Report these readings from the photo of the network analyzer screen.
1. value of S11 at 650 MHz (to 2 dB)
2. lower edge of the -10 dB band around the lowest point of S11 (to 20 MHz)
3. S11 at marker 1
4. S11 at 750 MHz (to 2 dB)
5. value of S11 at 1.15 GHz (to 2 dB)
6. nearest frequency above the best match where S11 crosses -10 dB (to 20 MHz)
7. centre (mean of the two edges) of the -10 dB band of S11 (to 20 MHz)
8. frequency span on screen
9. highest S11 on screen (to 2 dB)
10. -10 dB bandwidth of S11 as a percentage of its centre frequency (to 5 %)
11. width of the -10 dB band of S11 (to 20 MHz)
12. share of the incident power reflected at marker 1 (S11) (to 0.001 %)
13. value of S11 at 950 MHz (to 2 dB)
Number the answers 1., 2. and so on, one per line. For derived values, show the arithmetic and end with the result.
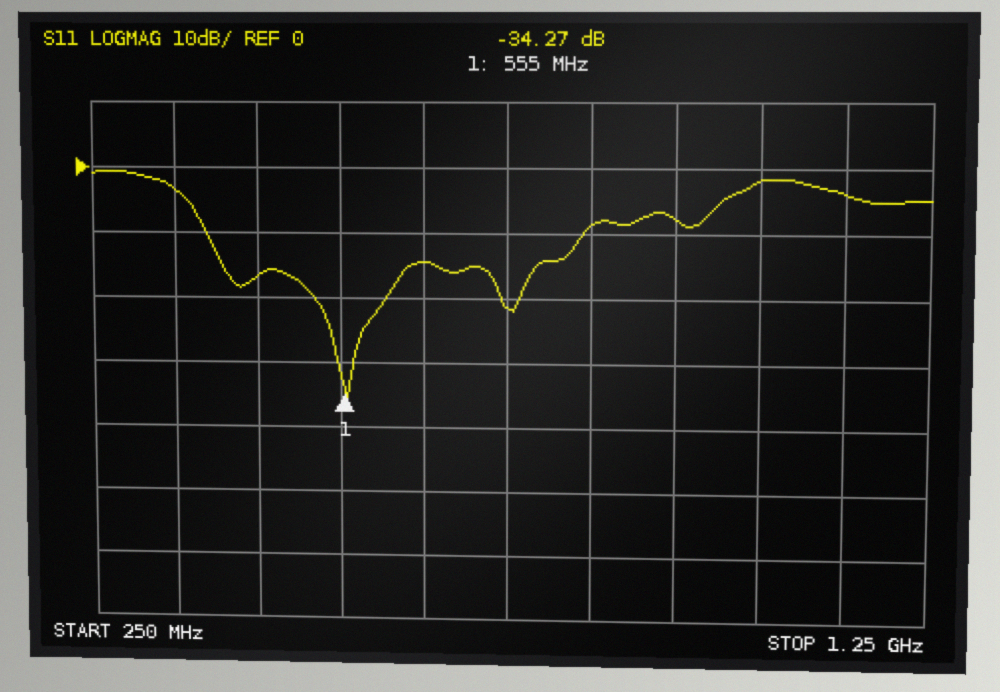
1. -14 dB
2. 380 MHz
3. -34.27 dB
4. -22 dB
5. -4 dB
6. 840 MHz
7. 620 MHz
8. 1 GHz
9. 0 dB
10. 460 MHz / 610 MHz ≈ 75 %
11. 840 MHz − 380 MHz = 460 MHz
12. 10^(-34.27/10) ≈ 0.037 %
13. -8 dB
